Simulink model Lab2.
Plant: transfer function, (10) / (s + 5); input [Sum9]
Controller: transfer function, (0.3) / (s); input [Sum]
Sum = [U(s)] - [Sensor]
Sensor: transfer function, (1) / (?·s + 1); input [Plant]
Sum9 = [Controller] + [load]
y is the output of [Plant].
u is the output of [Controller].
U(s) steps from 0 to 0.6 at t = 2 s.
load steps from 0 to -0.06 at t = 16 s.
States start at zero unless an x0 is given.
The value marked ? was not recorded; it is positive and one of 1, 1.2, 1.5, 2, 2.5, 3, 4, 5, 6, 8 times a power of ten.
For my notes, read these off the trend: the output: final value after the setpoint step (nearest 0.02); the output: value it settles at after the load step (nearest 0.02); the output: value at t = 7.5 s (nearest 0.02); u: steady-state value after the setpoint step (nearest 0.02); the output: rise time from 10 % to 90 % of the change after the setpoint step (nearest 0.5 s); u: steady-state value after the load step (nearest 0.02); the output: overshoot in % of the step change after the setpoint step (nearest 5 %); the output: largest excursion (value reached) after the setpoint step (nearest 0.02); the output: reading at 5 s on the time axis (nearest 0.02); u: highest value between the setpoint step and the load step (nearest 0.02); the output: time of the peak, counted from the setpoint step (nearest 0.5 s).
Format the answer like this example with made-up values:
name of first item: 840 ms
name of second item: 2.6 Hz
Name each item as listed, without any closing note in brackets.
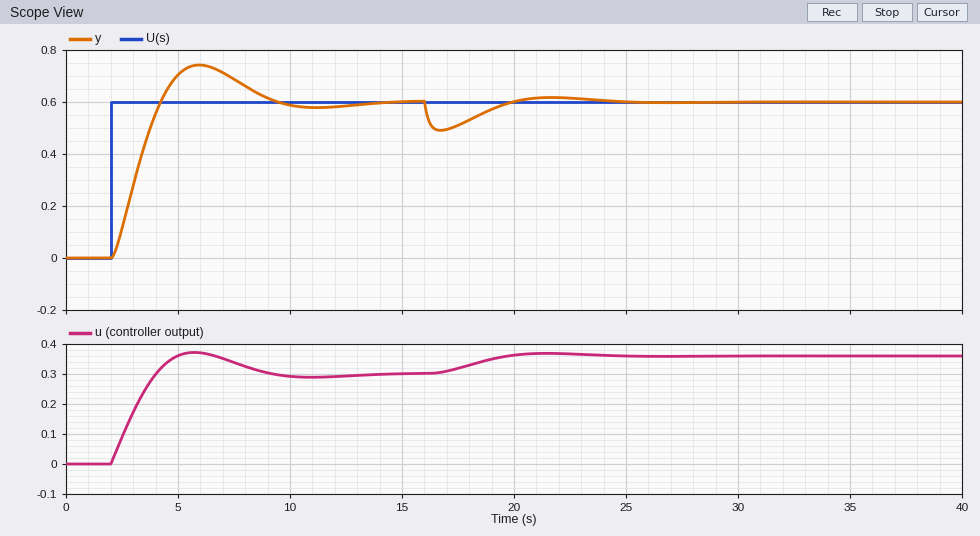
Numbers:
the output: final value after the setpoint step: 0.60
the output: value it settles at after the load step: 0.60
the output: value at t = 7.5 s: 0.68
u: steady-state value after the setpoint step: 0.30
the output: rise time from 10 % to 90 % of the change after the setpoint step: 1.5 s
u: steady-state value after the load step: 0.36
the output: overshoot in % of the step change after the setpoint step: 25 %
the output: largest excursion (value reached) after the setpoint step: 0.74
the output: reading at 5 s on the time axis: 0.70
u: highest value between the setpoint step and the load step: 0.38
the output: time of the peak, counted from the setpoint step: 4.0 s
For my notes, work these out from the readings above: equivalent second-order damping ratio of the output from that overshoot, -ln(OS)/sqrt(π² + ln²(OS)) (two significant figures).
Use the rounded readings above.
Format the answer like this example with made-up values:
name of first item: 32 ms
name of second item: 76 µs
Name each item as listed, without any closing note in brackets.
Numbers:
equivalent second-order damping ratio of the output from that overshoot, -ln(OS)/sqrt(π² + ln²(OS)): 0.40
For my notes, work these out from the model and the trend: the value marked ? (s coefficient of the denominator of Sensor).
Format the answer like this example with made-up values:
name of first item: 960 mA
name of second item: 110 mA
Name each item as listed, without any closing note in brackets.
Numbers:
the value marked ?: 1.2
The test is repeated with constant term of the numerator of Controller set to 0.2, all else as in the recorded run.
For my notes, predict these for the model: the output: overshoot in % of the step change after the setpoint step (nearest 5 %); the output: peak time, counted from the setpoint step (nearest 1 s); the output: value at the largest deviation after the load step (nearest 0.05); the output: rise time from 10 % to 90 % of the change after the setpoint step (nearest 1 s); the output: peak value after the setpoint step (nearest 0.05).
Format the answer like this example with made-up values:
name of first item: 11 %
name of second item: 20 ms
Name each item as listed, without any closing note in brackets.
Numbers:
the output: overshoot in % of the step change after the setpoint step: 10 %
the output: peak time, counted from the setpoint step: 6 s
the output: value at the largest deviation after the load step: 0.50
the output: rise time from 10 % to 90 % of the change after the setpoint step: 3 s
the output: peak value after the setpoint step: 0.65
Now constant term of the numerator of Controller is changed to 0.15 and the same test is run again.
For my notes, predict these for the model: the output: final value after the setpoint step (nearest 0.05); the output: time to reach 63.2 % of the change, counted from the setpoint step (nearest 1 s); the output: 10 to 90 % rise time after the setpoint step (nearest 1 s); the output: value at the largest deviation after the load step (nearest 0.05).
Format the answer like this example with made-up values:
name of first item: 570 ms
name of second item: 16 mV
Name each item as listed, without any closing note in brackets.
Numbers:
the output: final value after the setpoint step: 0.60
the output: time to reach 63.2 % of the change, counted from the setpoint step: 3 s
the output: 10 to 90 % rise time after the setpoint step: 4 s
the output: value at the largest deviation after the load step: 0.50
